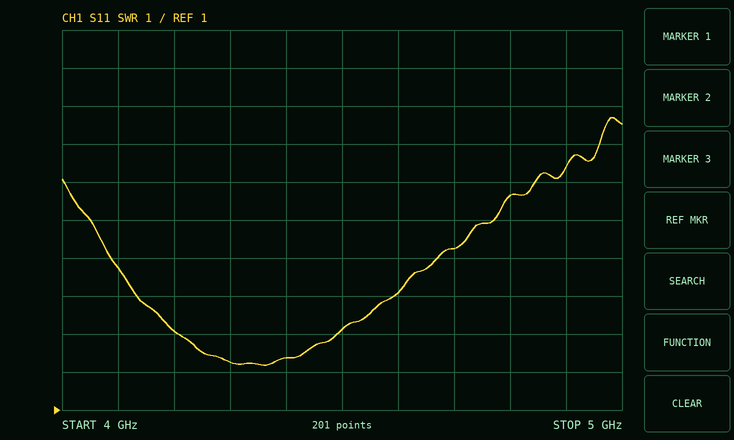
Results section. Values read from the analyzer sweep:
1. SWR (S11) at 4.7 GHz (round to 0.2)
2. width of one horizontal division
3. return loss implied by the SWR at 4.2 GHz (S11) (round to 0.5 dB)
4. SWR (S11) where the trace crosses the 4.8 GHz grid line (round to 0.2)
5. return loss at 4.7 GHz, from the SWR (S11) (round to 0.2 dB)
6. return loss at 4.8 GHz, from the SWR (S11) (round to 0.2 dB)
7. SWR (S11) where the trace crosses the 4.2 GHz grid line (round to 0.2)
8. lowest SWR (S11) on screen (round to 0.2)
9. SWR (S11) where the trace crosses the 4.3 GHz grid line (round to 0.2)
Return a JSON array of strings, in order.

["5.2", "100 MHz", "6.0 dB", "6.6", "3.4 dB", "2.6 dB", "3.0", "2.2", "2.2"]
